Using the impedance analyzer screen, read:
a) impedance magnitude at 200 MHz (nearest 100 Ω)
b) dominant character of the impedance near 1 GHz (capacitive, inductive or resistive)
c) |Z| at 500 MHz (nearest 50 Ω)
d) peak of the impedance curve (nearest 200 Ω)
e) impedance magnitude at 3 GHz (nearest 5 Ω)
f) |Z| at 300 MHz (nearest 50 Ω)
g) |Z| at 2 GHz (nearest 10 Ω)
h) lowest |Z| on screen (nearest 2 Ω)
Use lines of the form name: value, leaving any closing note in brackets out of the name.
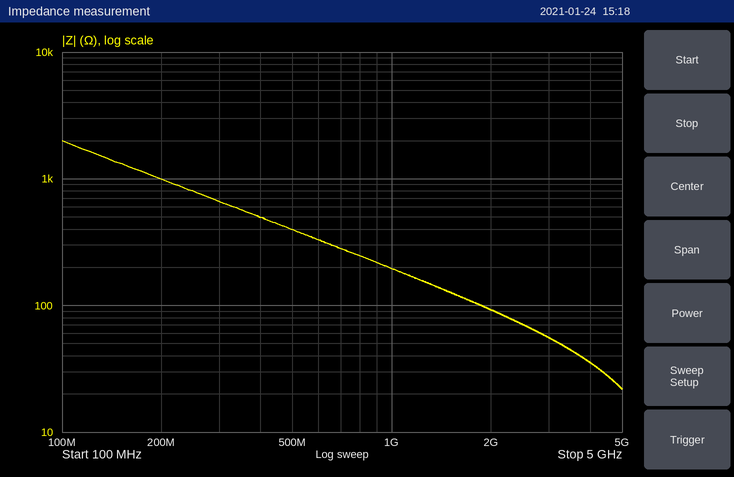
impedance magnitude at 200 MHz: 1.0 kΩ
dominant character of the impedance near 1 GHz: capacitive
|Z| at 500 MHz: 400 Ω
peak of the impedance curve: 2.0 kΩ
impedance magnitude at 3 GHz: 55 Ω
|Z| at 300 MHz: 650 Ω
|Z| at 2 GHz: 90 Ω
lowest |Z| on screen: 22 Ω
